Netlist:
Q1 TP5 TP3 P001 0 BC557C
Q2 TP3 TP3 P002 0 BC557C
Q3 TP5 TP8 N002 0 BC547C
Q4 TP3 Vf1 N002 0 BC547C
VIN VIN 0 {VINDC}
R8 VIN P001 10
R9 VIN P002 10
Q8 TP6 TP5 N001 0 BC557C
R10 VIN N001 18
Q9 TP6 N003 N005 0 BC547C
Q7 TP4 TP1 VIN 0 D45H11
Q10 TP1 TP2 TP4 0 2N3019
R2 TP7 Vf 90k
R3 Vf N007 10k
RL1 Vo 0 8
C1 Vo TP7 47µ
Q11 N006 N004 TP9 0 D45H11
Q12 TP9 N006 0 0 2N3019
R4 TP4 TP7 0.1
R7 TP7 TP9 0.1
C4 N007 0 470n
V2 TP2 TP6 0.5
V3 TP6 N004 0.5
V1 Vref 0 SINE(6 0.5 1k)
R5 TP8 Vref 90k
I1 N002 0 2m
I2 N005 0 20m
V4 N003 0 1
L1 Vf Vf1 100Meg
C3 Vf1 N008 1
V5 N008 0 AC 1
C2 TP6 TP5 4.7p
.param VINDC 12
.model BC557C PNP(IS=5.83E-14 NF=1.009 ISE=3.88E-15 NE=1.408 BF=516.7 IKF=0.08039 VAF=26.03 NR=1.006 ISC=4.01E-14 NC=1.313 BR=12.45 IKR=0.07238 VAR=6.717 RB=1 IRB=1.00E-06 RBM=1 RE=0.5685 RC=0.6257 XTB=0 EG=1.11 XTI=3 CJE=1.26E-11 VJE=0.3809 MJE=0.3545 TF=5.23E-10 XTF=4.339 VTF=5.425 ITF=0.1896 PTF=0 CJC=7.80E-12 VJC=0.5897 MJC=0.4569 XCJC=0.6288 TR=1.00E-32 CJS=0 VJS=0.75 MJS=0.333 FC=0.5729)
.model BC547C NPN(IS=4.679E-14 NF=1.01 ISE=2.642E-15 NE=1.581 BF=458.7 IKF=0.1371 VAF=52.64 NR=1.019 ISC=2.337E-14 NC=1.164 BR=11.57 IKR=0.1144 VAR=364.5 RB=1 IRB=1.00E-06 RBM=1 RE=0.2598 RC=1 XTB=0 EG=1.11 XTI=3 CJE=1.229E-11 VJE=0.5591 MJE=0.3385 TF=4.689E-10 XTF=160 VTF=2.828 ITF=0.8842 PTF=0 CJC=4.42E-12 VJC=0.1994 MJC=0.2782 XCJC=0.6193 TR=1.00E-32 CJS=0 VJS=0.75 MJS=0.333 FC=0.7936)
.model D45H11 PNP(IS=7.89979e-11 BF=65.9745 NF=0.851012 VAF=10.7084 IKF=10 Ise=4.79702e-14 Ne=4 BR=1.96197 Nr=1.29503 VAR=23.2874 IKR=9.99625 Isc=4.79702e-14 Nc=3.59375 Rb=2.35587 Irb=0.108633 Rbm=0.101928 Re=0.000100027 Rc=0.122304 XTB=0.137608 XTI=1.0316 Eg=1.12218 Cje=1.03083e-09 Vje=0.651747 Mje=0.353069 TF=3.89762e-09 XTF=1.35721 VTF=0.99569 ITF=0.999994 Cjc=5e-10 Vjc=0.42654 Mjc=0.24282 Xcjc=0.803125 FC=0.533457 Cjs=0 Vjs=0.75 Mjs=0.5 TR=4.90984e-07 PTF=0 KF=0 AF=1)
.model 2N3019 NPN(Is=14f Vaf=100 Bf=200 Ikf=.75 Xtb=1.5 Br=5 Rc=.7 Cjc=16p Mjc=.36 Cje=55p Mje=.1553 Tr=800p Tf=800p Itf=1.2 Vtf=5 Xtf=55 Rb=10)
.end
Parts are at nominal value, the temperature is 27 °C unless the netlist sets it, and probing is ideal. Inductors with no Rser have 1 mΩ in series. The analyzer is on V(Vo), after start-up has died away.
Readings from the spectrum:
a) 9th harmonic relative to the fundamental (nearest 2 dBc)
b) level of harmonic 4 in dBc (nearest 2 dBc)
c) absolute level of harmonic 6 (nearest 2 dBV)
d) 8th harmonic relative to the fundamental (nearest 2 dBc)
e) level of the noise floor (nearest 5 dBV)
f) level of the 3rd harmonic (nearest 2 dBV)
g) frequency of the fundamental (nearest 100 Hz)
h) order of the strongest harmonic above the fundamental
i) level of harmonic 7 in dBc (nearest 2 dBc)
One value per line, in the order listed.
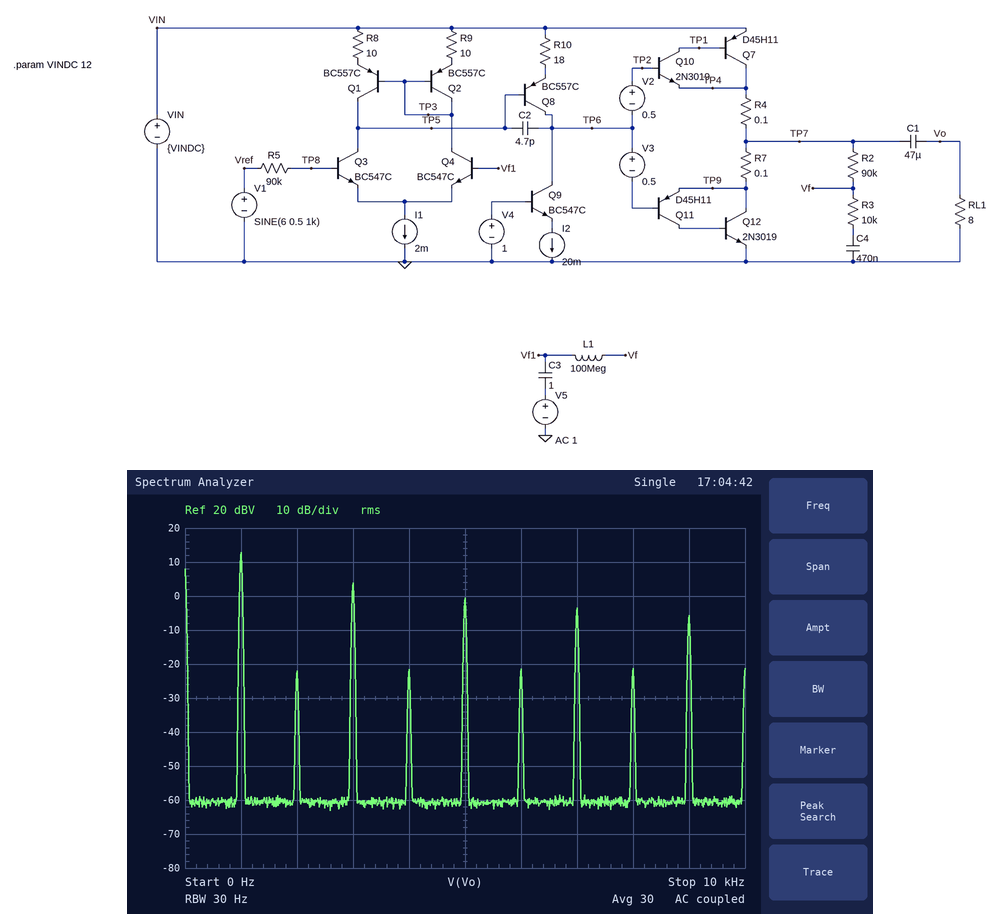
-18 dBc
-34 dBc
-22 dBV
-34 dBc
-60 dBV
4 dBV
1.0 kHz
3
-16 dBc
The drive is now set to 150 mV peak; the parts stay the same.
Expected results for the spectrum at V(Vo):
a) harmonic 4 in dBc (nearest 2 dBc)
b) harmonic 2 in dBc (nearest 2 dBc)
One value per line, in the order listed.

-32 dBc
-32 dBc
